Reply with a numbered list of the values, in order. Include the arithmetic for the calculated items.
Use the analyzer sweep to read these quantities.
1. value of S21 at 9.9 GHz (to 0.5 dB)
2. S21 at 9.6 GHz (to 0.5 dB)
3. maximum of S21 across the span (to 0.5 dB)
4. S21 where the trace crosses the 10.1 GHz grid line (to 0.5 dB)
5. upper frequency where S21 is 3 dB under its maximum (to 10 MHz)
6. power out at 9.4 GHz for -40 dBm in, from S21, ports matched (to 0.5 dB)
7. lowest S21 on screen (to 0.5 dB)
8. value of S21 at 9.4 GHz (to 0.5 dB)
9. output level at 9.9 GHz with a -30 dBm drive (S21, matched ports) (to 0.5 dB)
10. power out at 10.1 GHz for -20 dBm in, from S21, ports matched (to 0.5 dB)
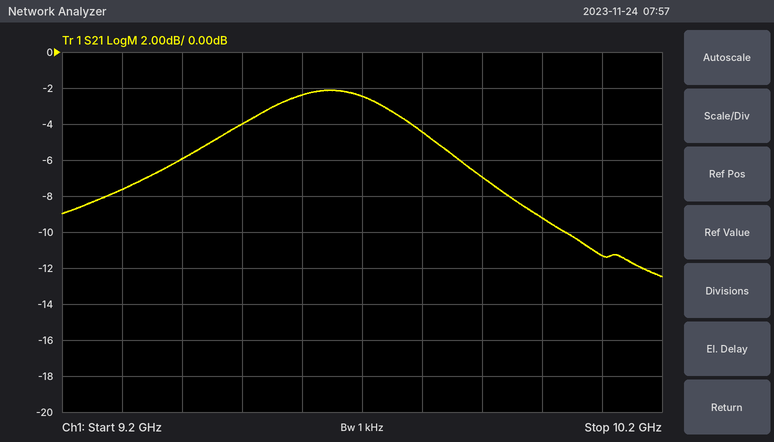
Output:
1. -7.0 dB
2. -2.5 dB
3. -2.0 dB
4. -11.5 dB
5. 9.83 GHz
6. -40 dBm + (-6.0 dB) = -46.0 dBm
7. -12.5 dB
8. -6.0 dB
9. -30 dBm + (-7.0 dB) = -37.0 dBm
10. -20 dBm + (-11.5 dB) = -31.5 dBm
